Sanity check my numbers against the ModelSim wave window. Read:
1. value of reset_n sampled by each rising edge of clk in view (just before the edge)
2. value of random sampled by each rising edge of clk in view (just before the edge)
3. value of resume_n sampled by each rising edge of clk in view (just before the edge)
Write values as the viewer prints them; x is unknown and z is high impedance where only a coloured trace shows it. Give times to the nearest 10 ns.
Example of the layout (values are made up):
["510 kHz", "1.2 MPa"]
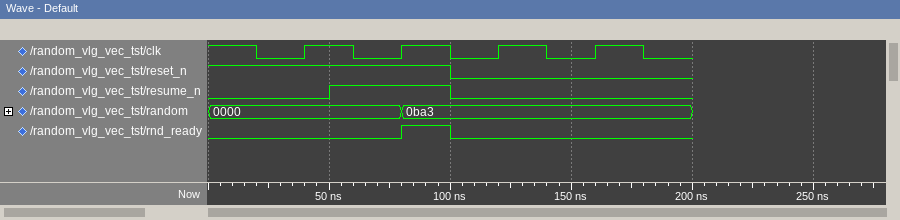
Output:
["1 1 0 0", "0000, 0000, 0ba3, 0ba3", "0 1 0 0"]
